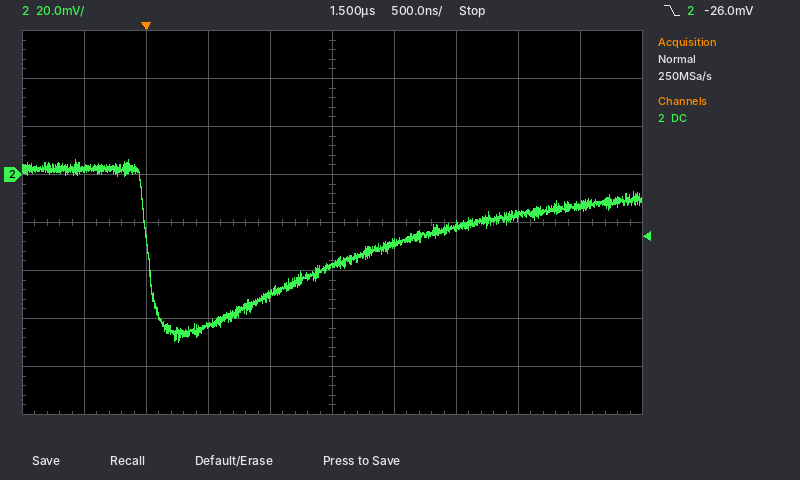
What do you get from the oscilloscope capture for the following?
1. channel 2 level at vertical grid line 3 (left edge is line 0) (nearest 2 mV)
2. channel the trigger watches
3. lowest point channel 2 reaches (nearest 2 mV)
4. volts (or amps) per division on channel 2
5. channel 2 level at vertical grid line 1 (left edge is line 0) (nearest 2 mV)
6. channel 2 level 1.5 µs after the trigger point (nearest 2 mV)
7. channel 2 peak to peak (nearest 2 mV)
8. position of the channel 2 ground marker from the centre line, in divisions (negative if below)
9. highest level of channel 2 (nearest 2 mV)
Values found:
-62 mV
channel 2
-70 mV
20 mV
2 mV
-38 mV
76 mV
+1.0 div
6 mV
